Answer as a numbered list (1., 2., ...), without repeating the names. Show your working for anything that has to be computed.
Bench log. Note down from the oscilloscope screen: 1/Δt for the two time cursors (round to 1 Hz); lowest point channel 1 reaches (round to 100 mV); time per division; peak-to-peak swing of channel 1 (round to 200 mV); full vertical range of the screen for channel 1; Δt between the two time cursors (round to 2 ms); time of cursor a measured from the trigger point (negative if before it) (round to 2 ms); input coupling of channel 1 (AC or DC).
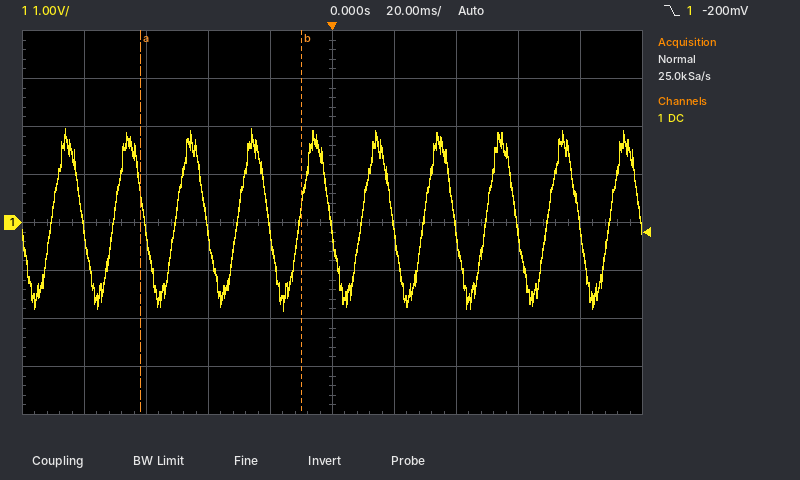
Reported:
1. 1 / 52 ms ≈ 19 Hz
2. -1.8 V
3. 20 ms
4. 3.8 V
5. 8 V
6. 52 ms
7. -62 ms
8. DC
